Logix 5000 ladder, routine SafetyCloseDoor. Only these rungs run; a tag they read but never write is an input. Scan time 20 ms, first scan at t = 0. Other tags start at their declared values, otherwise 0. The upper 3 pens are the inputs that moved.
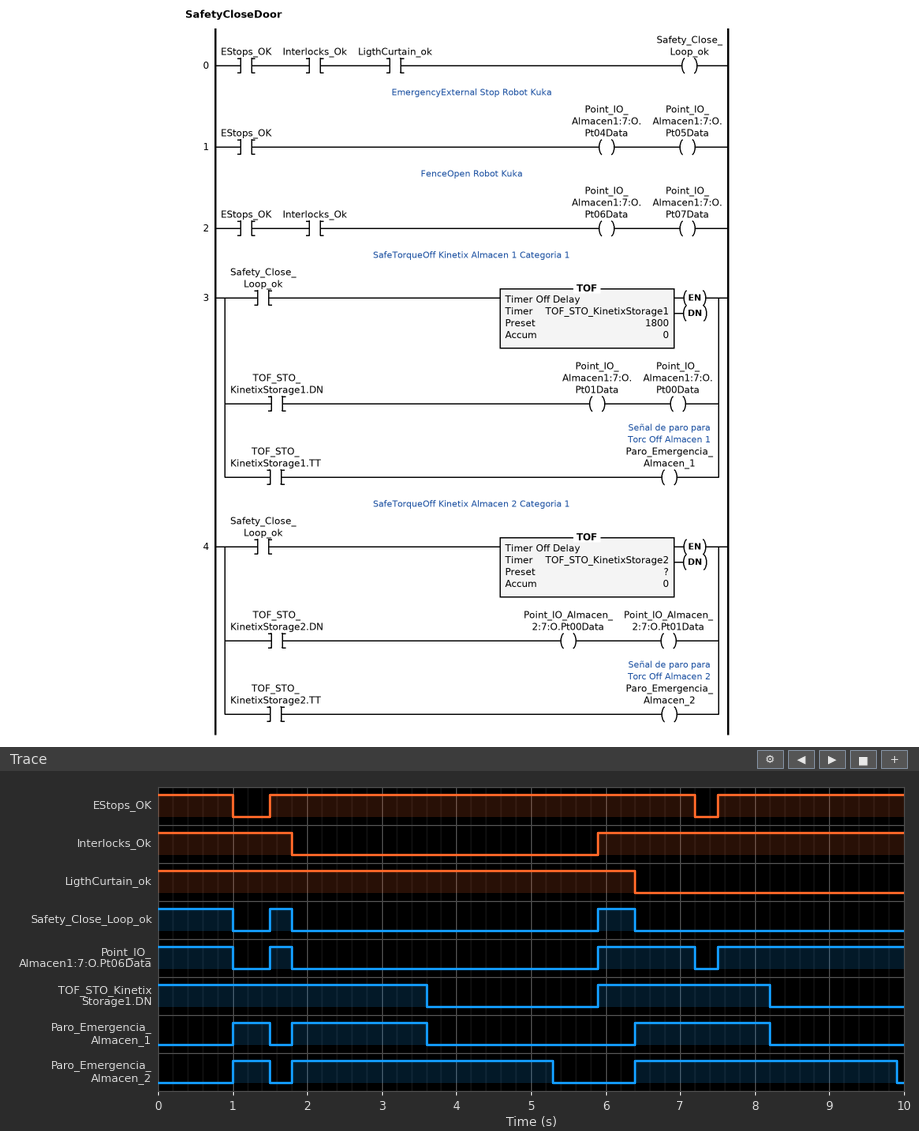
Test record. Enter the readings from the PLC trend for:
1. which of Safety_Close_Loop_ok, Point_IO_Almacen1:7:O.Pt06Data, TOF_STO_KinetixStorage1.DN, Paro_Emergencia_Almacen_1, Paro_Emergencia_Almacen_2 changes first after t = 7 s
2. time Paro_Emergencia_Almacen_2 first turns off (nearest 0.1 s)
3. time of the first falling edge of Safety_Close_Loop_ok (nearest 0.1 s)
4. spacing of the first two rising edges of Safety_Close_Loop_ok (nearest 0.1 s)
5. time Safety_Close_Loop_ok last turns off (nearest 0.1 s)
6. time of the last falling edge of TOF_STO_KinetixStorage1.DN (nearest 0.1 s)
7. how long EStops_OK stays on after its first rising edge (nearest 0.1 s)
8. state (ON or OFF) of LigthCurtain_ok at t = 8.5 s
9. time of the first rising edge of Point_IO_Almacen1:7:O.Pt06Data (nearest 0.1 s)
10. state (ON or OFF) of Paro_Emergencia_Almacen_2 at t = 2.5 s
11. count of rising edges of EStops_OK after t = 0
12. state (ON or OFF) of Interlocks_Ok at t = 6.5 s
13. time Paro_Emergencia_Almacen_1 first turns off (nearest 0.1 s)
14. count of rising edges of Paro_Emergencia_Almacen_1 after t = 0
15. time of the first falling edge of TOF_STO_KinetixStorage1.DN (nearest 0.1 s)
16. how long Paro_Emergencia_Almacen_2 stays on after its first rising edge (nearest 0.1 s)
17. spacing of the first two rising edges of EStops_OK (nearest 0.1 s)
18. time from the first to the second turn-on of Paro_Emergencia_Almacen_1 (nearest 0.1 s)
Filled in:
Point_IO_Almacen1:7:O.Pt06Data
1.5 s
1.0 s
4.4 s
6.4 s
8.2 s
5.7 s
OFF
1.5 s
ON
2
ON
1.5 s
3
3.6 s
0.5 s
6.0 s
0.8 s
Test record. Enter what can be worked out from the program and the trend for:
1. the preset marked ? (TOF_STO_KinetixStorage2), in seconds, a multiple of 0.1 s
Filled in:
3.5 s
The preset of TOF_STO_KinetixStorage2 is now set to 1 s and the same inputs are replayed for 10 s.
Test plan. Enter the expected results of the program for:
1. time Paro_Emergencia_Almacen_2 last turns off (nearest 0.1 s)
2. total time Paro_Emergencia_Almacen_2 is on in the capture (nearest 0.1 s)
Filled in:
7.4 s
2.5 s
